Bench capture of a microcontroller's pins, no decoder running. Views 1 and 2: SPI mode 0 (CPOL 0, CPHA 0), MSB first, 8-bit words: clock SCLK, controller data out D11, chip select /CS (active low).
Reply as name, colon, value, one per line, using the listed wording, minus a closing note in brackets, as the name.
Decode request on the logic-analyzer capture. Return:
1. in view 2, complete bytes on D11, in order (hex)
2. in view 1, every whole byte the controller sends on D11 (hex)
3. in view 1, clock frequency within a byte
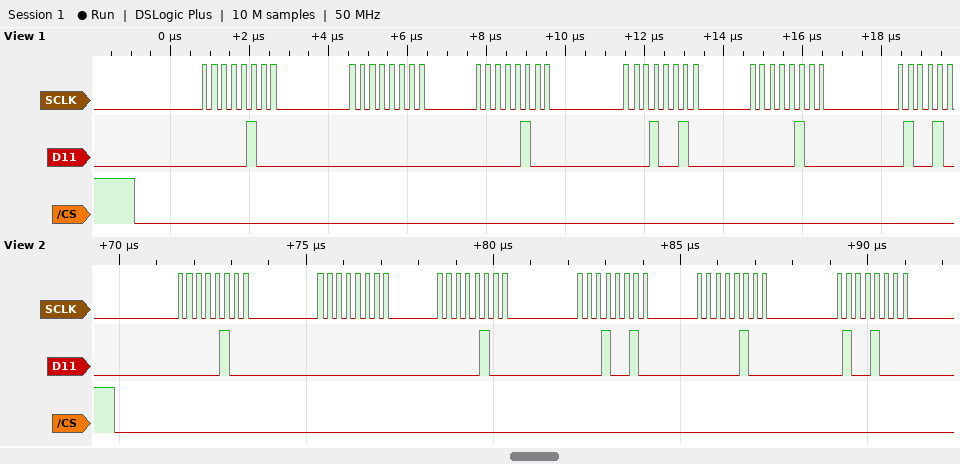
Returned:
in view 2, complete bytes on D11, in order: 04 00 04 12 04 48
in view 1, every whole byte the controller sends on D11: 0x04 0x00 0x04 0x12 0x04
in view 1, clock frequency within a byte: 4 MHz
